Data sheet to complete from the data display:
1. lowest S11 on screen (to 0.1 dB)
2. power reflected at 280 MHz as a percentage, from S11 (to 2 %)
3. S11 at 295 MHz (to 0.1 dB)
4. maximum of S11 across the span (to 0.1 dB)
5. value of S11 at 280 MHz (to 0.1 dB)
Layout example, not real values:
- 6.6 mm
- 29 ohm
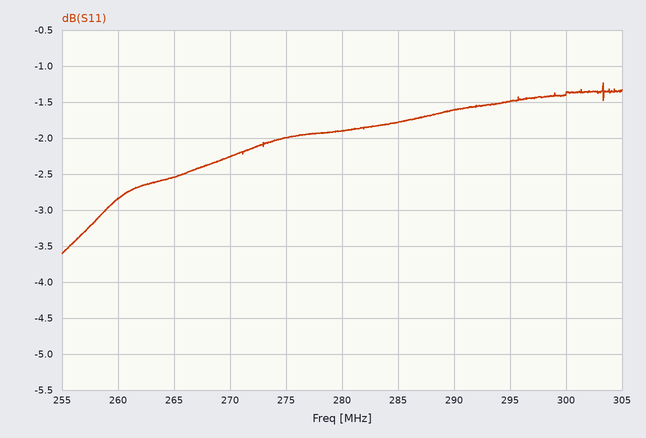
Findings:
- -3.6 dB
- 64 %
- -1.5 dB
- -1.2 dB
- -1.9 dB
